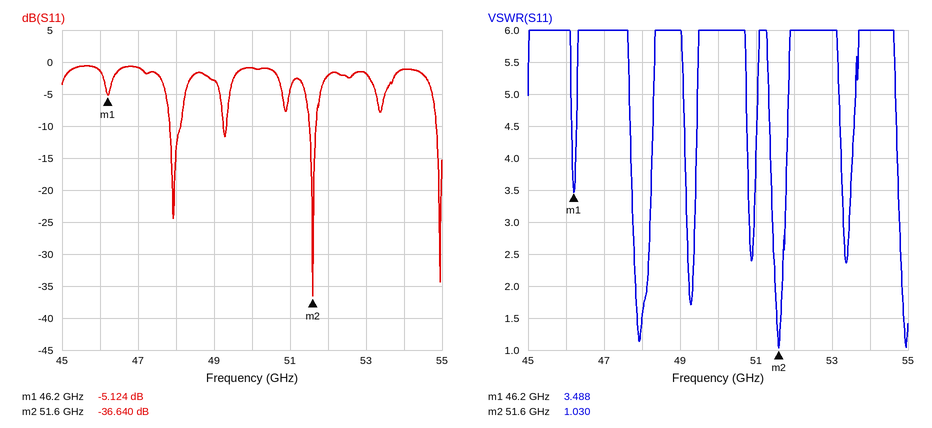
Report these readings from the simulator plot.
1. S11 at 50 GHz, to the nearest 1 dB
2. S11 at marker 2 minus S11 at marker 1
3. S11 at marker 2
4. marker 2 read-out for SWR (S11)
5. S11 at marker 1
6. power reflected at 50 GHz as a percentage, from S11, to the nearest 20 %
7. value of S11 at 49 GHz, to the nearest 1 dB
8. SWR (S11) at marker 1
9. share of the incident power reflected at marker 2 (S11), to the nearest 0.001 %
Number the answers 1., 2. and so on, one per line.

1. -1 dB
2. -31.516 dB
3. -36.640 dB
4. 1.030
5. -5.124 dB
6. 80 %
7. -3 dB
8. 3.488
9. 0.022 %
